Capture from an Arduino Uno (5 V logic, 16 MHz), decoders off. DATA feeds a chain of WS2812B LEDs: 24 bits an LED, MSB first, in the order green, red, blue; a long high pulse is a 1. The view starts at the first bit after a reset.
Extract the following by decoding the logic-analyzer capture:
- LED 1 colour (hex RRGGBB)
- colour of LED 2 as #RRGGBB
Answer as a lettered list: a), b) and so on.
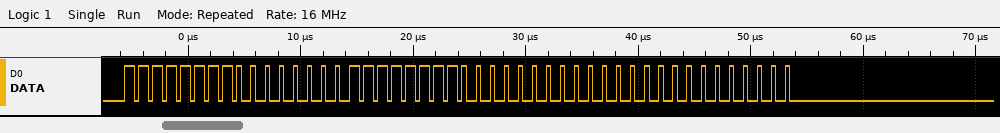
a) #00FFFF
b) #000000
